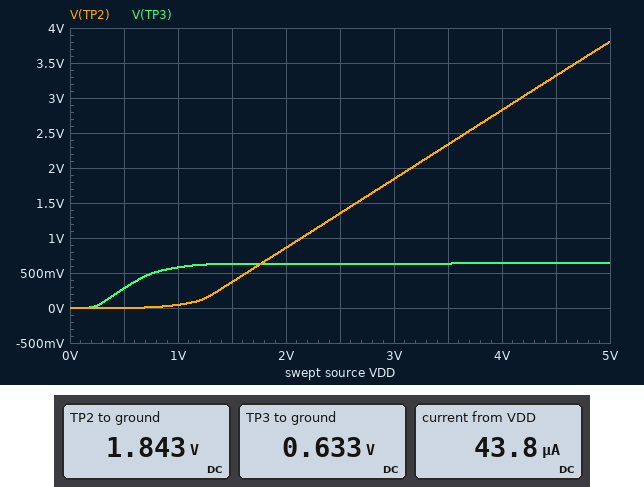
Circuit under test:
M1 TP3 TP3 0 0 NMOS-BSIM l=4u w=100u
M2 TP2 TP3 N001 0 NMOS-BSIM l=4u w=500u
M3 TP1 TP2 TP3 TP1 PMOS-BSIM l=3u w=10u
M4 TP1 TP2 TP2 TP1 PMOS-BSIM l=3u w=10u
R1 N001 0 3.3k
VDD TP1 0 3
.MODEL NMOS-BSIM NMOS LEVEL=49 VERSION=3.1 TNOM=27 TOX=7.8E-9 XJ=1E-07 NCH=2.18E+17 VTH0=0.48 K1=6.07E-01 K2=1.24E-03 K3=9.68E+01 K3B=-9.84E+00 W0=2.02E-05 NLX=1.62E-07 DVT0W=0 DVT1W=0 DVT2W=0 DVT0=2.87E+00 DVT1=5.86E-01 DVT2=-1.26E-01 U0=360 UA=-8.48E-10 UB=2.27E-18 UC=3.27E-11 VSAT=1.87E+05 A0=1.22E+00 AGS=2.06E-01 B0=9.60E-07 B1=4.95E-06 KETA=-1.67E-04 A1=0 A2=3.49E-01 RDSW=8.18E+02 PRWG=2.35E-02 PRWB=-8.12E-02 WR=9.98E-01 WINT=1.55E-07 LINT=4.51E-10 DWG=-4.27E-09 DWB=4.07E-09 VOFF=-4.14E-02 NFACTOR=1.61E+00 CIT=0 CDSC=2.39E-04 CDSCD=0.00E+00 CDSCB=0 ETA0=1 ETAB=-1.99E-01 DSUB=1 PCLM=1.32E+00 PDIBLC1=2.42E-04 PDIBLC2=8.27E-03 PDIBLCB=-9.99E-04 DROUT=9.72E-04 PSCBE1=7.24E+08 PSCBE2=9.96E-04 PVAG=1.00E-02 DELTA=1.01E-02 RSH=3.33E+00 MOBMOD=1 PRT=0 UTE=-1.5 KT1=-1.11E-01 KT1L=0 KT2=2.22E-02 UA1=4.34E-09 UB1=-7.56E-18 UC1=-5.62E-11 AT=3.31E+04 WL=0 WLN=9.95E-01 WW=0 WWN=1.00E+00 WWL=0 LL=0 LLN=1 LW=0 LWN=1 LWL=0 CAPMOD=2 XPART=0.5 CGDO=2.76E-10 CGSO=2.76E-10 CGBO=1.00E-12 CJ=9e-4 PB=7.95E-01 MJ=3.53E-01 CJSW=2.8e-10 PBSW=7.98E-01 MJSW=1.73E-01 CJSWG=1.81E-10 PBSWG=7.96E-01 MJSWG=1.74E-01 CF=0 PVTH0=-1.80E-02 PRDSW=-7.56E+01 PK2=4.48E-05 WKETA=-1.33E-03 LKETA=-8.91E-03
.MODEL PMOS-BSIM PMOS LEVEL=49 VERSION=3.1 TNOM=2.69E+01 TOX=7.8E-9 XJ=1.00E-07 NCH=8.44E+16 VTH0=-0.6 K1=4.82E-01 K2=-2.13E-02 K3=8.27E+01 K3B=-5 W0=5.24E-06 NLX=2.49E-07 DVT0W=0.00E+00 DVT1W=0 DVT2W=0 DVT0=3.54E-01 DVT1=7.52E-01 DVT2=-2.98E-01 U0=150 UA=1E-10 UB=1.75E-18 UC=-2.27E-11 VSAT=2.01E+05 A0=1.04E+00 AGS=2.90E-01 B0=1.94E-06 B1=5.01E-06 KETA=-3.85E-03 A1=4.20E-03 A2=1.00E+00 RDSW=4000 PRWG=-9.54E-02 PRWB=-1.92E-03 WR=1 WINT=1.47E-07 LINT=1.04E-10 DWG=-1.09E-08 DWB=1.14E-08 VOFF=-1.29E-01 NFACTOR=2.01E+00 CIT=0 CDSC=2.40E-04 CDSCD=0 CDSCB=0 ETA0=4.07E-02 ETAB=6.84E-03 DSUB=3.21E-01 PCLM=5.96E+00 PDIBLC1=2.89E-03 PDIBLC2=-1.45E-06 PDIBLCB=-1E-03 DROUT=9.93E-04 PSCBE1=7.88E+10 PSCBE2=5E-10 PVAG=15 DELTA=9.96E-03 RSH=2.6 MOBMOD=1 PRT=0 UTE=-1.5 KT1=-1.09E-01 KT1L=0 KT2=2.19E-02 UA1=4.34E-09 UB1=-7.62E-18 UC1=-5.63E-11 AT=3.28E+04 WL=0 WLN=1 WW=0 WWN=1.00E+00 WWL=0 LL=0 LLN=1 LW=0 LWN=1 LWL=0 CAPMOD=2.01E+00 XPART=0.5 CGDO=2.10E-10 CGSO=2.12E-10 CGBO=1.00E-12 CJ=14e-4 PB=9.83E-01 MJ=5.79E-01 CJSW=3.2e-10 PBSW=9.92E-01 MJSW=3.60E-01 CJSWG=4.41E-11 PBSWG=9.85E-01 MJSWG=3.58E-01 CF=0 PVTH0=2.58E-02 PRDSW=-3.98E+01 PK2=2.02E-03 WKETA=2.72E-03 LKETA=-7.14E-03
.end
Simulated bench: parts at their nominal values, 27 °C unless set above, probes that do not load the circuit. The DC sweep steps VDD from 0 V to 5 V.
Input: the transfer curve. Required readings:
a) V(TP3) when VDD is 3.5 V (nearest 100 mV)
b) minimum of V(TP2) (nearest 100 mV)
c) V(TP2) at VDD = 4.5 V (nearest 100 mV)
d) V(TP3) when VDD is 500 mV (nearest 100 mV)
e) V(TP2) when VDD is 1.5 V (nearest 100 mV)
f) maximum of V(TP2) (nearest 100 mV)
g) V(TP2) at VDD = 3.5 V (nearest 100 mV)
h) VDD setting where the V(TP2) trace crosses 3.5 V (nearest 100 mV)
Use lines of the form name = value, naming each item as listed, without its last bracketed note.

V(TP3) when VDD is 3.5 V = 600 mV
minimum of V(TP2) = 0 V
V(TP2) at VDD = 4.5 V = 3.3 V
V(TP3) when VDD is 500 mV = 300 mV
V(TP2) when VDD is 1.5 V = 400 mV
maximum of V(TP2) = 3.8 V
V(TP2) at VDD = 3.5 V = 2.3 V
VDD setting where the V(TP2) trace crosses 3.5 V = 4.7 V
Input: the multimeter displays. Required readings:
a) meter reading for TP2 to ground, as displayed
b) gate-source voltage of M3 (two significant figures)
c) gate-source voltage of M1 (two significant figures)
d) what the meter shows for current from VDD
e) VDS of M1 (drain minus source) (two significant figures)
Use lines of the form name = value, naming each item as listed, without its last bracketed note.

meter reading for TP2 to ground, as displayed = 1.843 V
gate-source voltage of M3 = 1.2 V
gate-source voltage of M1 = 630 mV
what the meter shows for current from VDD = 43.8 µA
VDS of M1 (drain minus source) = 630 mV
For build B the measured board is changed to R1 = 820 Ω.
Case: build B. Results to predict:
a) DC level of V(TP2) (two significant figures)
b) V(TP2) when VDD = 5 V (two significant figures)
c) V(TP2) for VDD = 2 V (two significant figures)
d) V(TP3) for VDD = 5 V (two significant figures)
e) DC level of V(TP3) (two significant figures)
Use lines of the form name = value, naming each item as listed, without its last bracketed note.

DC level of V(TP2) = 970 mV
V(TP2) when VDD = 5 V = 2.9 V
V(TP2) for VDD = 2 V = 160 mV
V(TP3) for VDD = 5 V = 810 mV
DC level of V(TP3) = 790 mV
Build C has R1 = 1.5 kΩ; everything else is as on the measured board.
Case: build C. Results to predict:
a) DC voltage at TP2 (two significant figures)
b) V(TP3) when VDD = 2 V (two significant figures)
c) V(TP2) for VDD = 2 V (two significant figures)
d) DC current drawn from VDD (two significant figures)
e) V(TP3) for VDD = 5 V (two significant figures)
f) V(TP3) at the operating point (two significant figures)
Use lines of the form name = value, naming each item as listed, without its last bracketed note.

DC voltage at TP2 = 1.5 V
V(TP3) when VDD = 2 V = 690 mV
V(TP2) for VDD = 2 V = 530 mV
DC current drawn from VDD = 110 µA
V(TP3) for VDD = 5 V = 710 mV
V(TP3) at the operating point = 700 mV
